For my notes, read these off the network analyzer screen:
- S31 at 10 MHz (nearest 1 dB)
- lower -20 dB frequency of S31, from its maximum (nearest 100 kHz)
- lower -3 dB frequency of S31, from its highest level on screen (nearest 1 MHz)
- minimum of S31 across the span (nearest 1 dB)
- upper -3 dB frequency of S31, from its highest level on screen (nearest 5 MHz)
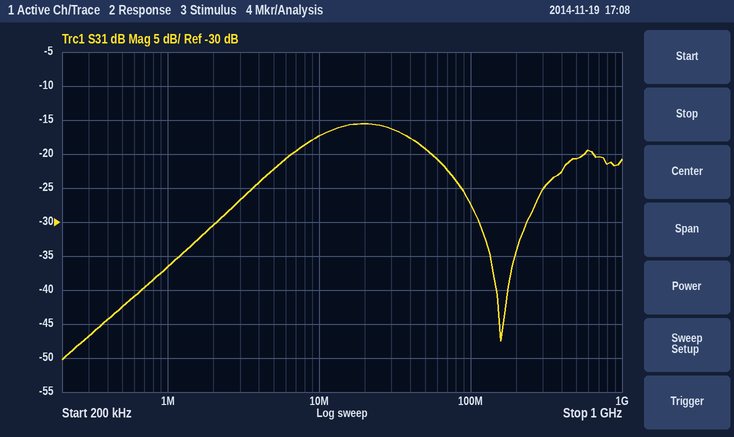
-17 dB
1.1 MHz
8 MHz
-50 dB
45 MHz
